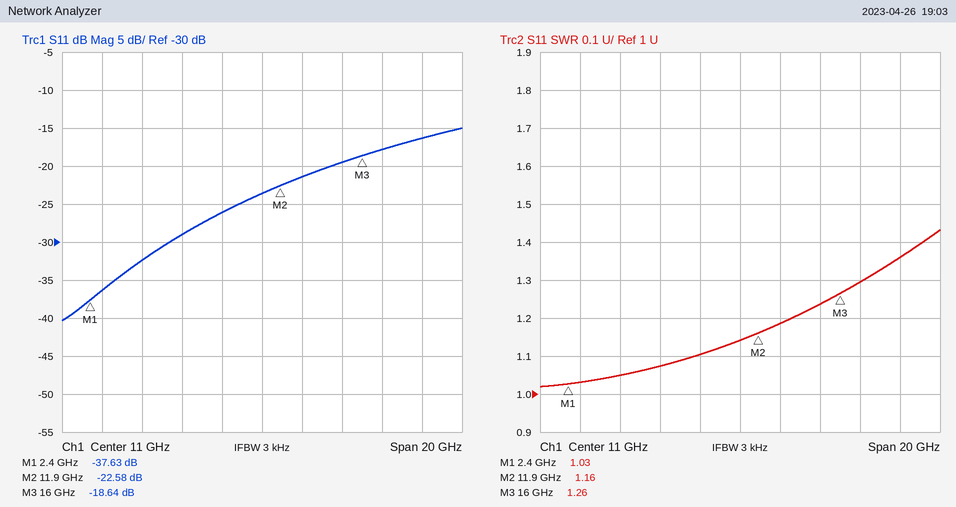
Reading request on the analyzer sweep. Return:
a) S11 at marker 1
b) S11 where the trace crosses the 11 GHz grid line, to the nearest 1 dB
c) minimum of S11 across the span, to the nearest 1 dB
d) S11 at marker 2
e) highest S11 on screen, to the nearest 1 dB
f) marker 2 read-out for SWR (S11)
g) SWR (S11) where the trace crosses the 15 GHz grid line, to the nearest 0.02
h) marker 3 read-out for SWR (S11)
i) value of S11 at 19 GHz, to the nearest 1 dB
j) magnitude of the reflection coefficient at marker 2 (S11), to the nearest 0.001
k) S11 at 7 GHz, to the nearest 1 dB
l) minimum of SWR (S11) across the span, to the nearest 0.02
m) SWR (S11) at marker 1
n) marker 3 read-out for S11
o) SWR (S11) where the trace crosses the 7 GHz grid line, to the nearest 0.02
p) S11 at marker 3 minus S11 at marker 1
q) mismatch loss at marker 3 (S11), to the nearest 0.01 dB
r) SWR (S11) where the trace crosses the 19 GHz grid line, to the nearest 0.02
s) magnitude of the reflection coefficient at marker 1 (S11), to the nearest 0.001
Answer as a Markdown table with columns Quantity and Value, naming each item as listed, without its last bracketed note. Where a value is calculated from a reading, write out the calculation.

| Quantity | Value |
|---|---|
| S11 at marker 1 | -37.63 dB |
| S11 where the trace crosses the 11 GHz grid line, to the nearest 1 dB | -24 dB |
| minimum of S11 across the span, to the nearest 1 dB | -40 dB |
| S11 at marker 2 | -22.58 dB |
| highest S11 on screen, to the nearest 1 dB | -15 dB |
| marker 2 read-out for SWR | 1.16 |
| SWR (S11) where the trace crosses the 15 GHz grid line, to the nearest 0.02 | 1.24 |
| marker 3 read-out for SWR | 1.26 |
| value of S11 at 19 GHz, to the nearest 1 dB | -16 dB |
| magnitude of the reflection coefficient at marker 2 (S11), to the nearest 0.001 | 10^(-22.58/20) ≈ 0.074 |
| S11 at 7 GHz, to the nearest 1 dB | -29 dB |
| minimum of SWR (S11) across the span, to the nearest 0.02 | 1.02 |
| SWR (S11) at marker 1 | 1.03 |
| marker 3 read-out for S11 | -18.64 dB |
| SWR (S11) where the trace crosses the 7 GHz grid line, to the nearest 0.02 | 1.08 |
| S11 at marker 3 minus S11 at marker 1 | -18.64 − (-37.63) = 18.99 dB |
| mismatch loss at marker 3 (S11), to the nearest 0.01 dB | −10 log10(1 − 10^(-18.64/10)) ≈ 0.06 dB |
| SWR (S11) where the trace crosses the 19 GHz grid line, to the nearest 0.02 | 1.36 |
| magnitude of the reflection coefficient at marker 1 (S11), to the nearest 0.001 | 10^(-37.63/20) ≈ 0.013 |
